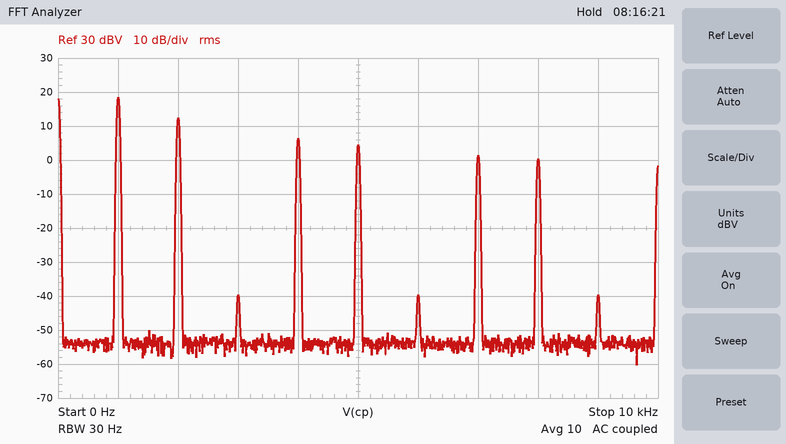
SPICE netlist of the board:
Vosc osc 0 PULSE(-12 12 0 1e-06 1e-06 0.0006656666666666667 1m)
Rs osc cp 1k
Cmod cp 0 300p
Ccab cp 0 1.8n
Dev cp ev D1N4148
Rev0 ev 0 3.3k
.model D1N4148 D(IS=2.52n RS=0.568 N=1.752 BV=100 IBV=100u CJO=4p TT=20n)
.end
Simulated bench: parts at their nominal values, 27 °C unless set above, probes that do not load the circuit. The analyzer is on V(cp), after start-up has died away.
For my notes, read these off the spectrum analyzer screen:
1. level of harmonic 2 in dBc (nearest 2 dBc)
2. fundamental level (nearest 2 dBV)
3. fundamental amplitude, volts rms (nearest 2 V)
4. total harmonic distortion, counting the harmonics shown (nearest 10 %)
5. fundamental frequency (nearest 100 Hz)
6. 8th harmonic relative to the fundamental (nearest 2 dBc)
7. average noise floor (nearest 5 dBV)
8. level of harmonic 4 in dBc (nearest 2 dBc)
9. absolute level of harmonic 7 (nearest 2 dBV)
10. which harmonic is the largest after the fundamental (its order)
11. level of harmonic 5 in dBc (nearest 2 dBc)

-6 dBc
18 dBV
8 V
60 %
1.0 kHz
-18 dBc
-55 dBV
-12 dBc
2 dBV
2
-14 dBc
